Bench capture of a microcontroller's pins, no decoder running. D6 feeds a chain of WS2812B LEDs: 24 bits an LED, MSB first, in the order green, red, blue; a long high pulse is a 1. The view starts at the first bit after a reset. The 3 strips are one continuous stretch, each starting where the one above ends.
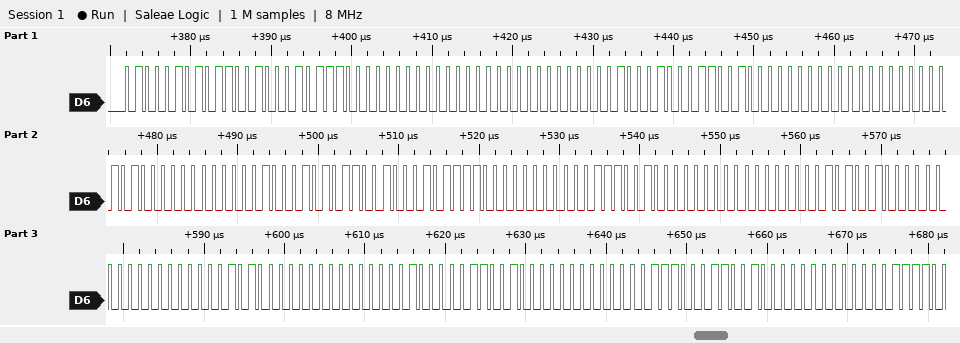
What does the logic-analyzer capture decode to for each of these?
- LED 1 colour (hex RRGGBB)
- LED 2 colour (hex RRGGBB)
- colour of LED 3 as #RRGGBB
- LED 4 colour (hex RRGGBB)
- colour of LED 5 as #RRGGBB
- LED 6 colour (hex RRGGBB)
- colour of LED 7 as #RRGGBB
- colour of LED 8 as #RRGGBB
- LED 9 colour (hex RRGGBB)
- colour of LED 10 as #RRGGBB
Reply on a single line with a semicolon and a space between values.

#64455C; #000000; #644400; #280000; #64455E; #390000; #520000; #500000; #641000; #641C00
